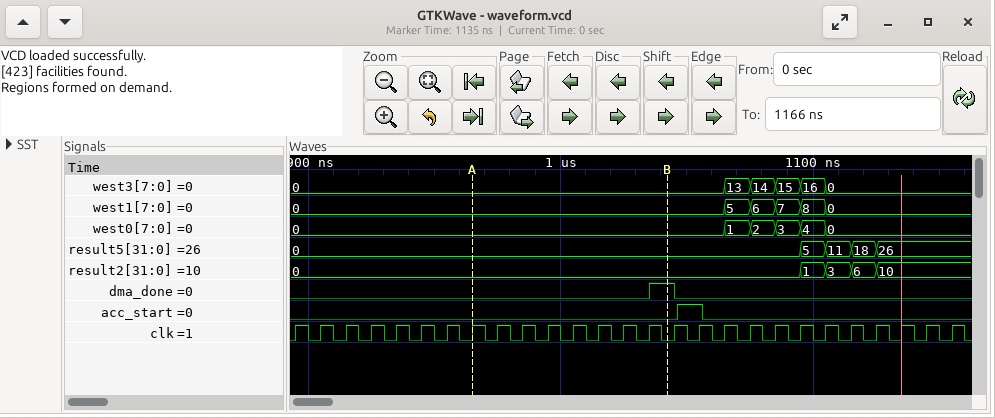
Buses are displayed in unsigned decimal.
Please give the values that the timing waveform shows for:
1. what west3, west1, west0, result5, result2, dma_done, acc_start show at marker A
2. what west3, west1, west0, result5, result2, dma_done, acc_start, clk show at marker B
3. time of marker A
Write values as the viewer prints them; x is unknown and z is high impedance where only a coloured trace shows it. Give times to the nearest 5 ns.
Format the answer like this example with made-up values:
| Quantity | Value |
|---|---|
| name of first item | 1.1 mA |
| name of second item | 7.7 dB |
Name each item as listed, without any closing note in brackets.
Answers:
| Quantity | Value |
|---|---|
| what west3, west1, west0, result5, result2, dma_done, acc_start show at marker A | west3=0, west1=0, west0=0, result5=0, result2=0, dma_done=0, acc_start=0 |
| what west3, west1, west0, result5, result2, dma_done, acc_start, clk show at marker B | west3=0, west1=0, west0=0, result5=0, result2=0, dma_done=1, acc_start=0, clk=0 |
| time of marker A | 965 ns |
